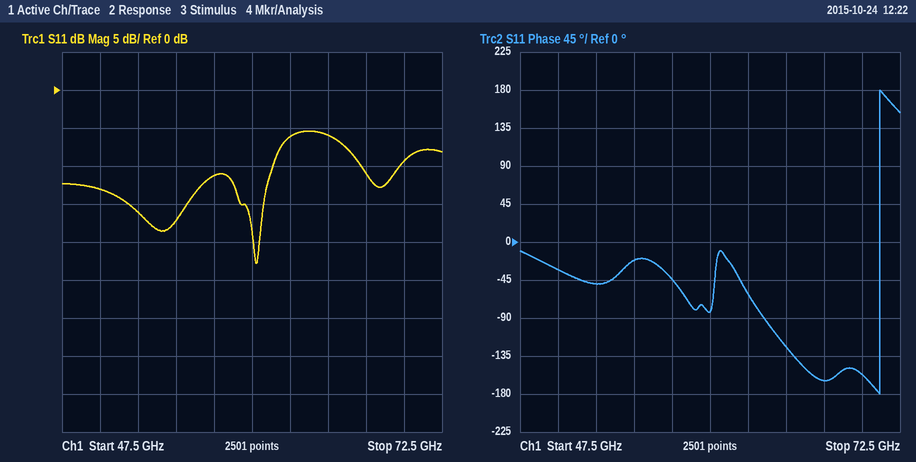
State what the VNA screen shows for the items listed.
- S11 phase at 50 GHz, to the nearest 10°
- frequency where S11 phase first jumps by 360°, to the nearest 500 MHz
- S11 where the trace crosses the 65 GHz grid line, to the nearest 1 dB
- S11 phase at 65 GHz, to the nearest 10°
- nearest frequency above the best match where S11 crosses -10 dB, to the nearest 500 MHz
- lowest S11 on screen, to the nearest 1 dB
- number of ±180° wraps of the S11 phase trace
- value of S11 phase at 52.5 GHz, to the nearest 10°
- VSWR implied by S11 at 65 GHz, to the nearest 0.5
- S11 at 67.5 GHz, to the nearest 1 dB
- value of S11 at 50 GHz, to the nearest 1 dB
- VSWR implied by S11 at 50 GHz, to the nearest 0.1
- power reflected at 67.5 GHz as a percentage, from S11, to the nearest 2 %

-30°
71.0 GHz
-6 dB
-120°
61.5 GHz
-23 dB
1
-50°
3.0
-11 dB
-13 dB
1.6
8 %
